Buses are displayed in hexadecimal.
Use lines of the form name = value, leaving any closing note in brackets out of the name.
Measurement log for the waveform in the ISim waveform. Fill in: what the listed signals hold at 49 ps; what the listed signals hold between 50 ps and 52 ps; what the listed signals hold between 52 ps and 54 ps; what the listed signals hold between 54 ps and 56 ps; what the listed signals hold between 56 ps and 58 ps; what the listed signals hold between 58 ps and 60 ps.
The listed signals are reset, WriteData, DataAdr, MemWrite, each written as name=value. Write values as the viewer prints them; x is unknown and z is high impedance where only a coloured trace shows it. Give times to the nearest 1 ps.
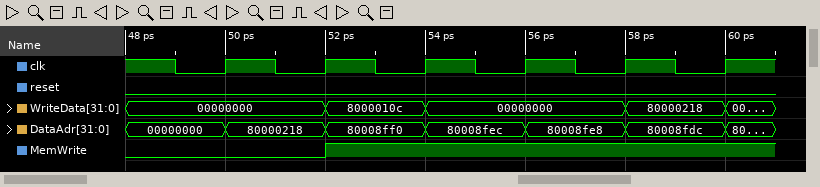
what the listed signals hold at 49 ps = reset=0, WriteData=00000000, DataAdr=00000000, MemWrite=0
what the listed signals hold between 50 ps and 52 ps = reset=0, WriteData=00000000, DataAdr=80000218, MemWrite=0
what the listed signals hold between 52 ps and 54 ps = reset=0, WriteData=8000010c, DataAdr=80008ff0, MemWrite=1
what the listed signals hold between 54 ps and 56 ps = reset=0, WriteData=00000000, DataAdr=80008fec, MemWrite=1
what the listed signals hold between 56 ps and 58 ps = reset=0, WriteData=00000000, DataAdr=80008fe8, MemWrite=1
what the listed signals hold between 58 ps and 60 ps = reset=0, WriteData=80000218, DataAdr=80008fdc, MemWrite=1
